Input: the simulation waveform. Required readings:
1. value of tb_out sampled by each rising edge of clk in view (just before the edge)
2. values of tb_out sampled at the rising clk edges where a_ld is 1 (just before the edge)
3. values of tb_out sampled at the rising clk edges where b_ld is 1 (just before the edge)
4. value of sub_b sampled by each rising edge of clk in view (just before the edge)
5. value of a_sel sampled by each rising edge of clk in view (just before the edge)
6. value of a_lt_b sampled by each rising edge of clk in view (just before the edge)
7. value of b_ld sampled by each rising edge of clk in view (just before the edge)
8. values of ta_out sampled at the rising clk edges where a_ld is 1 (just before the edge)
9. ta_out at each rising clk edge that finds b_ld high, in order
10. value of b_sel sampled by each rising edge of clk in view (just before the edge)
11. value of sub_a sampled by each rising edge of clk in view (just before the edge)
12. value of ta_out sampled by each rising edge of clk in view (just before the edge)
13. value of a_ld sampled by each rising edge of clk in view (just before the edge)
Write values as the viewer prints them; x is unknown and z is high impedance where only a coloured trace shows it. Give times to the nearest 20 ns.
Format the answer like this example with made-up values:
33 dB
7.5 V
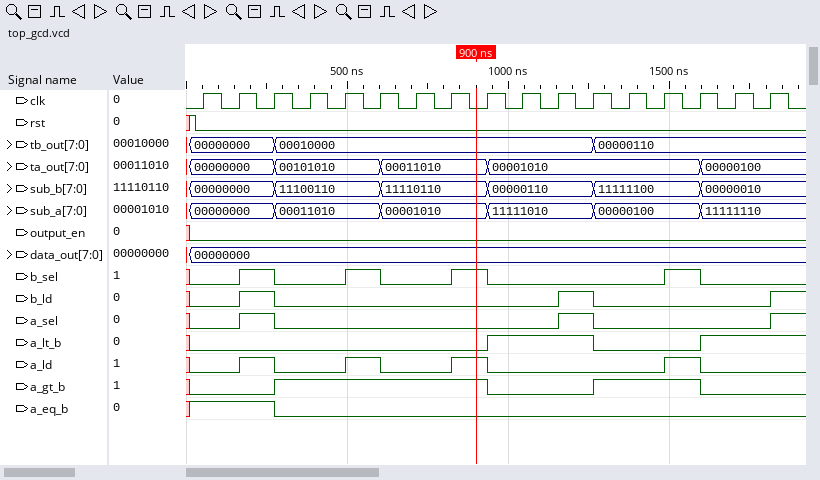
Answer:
00000000, 00000000, 00000000, 00010000, 00010000, 00010000, 00010000, 00010000, 00010000, 00010000, 00010000, 00010000, 00000110, 00000110, 00000110, 00000110, 00000110
00000000, 00010000, 00010000, 00000110
00000000, 00010000
00000000, 00000000, 00000000, 11100110, 11100110, 11100110, 11110110, 11110110, 11110110, 00000110, 00000110, 00000110, 11111100, 11111100, 11111100, 00000010, 00000010
0 0 1 0 0 0 0 0 0 0 0 1 0 0 0 0 0
0 0 0 0 0 0 0 0 0 1 1 1 0 0 0 1 1
0 0 1 0 0 0 0 0 0 0 0 1 0 0 0 0 0
00000000, 00101010, 00011010, 00001010
00000000, 00001010
0 0 1 0 0 1 0 0 1 0 0 0 0 0 1 0 0
00000000, 00000000, 00000000, 00011010, 00011010, 00011010, 00001010, 00001010, 00001010, 11111010, 11111010, 11111010, 00000100, 00000100, 00000100, 11111110, 11111110
00000000, 00000000, 00000000, 00101010, 00101010, 00101010, 00011010, 00011010, 00011010, 00001010, 00001010, 00001010, 00001010, 00001010, 00001010, 00000100, 00000100
0 0 1 0 0 1 0 0 1 0 0 0 0 0 1 0 0
